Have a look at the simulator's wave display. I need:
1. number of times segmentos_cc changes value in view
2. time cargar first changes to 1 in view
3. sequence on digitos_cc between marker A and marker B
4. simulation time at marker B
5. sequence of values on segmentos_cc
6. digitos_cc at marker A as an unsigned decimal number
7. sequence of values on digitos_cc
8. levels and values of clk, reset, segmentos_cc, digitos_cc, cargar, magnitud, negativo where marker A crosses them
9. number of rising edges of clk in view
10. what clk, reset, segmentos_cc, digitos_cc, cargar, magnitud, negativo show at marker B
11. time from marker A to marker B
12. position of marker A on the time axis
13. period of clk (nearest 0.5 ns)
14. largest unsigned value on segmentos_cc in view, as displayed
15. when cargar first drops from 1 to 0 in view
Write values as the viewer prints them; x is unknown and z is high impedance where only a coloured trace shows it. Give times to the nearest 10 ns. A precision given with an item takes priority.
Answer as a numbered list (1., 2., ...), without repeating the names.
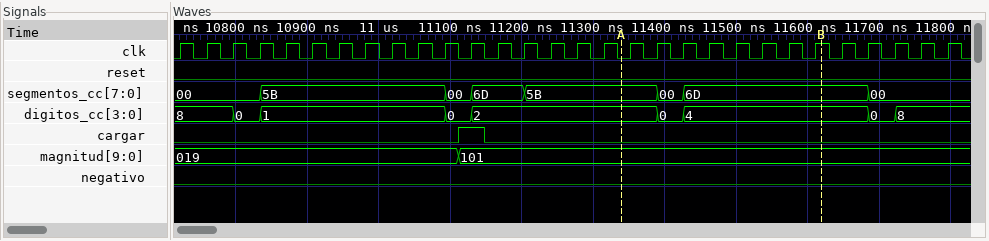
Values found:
1. 7
2. 11110 ns
3. 2, 0, 4
4. 11620 ns
5. 00, 5B, 00, 6D, 5B, 00, 6D, 00
6. 2
7. 8, 0, 1, 0, 2, 0, 4, 0, 8
8. clk=0, reset=0, segmentos_cc=5B, digitos_cc=2, cargar=0, magnitud=101, negativo=0
9. 30
10. clk=1, reset=0, segmentos_cc=6D, digitos_cc=4, cargar=0, magnitud=101, negativo=0
11. 280 ns
12. 11340 ns
13. 37 ns
14. 6D
15. 11150 ns
